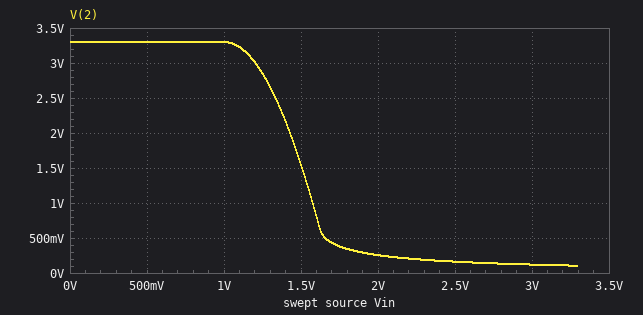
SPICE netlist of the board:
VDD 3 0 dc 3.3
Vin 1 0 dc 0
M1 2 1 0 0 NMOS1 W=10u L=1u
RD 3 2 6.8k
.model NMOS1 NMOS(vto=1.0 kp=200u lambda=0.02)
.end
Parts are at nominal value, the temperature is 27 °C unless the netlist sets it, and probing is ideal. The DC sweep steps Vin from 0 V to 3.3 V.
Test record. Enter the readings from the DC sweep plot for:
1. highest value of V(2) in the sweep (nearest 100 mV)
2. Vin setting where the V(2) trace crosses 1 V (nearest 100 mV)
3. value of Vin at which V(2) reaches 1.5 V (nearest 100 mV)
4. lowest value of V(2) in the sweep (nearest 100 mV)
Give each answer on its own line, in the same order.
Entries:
3.3 V
1.6 V
1.5 V
100 mV
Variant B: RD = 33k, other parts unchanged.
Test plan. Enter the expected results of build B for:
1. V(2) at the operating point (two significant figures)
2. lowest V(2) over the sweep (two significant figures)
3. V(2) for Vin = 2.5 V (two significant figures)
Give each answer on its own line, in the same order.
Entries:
3.3 V
22 mV
33 mV
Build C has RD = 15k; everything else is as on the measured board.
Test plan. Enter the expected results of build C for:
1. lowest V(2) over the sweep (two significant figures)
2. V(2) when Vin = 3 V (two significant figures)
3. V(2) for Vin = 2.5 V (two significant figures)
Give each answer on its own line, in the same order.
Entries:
48 mV
55 mV
73 mV
